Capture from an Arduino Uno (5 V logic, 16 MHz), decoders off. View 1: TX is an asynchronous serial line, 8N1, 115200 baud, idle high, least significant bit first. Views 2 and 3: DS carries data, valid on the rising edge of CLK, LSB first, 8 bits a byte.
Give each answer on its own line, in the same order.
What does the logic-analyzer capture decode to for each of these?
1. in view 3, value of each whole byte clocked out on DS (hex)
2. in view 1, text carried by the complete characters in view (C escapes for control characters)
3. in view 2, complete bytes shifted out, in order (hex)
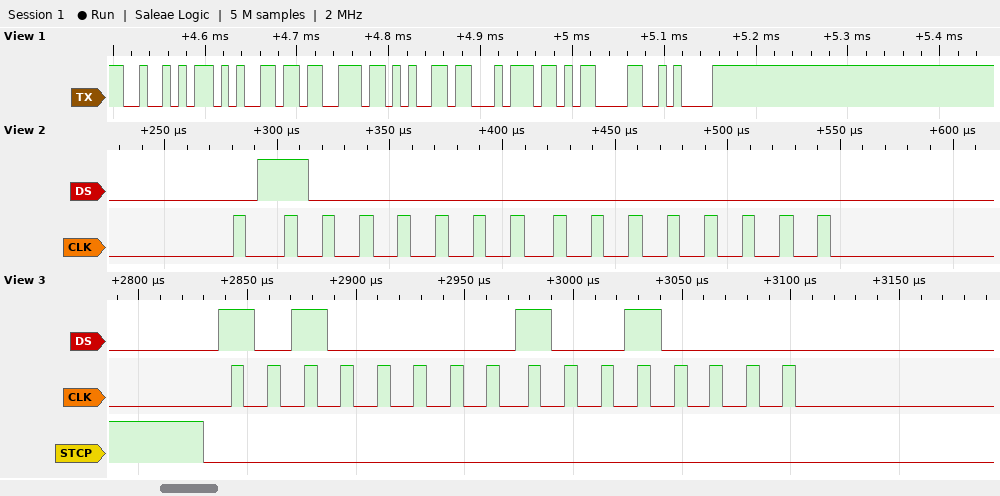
05 09
"Reset\r\n"
02 00
